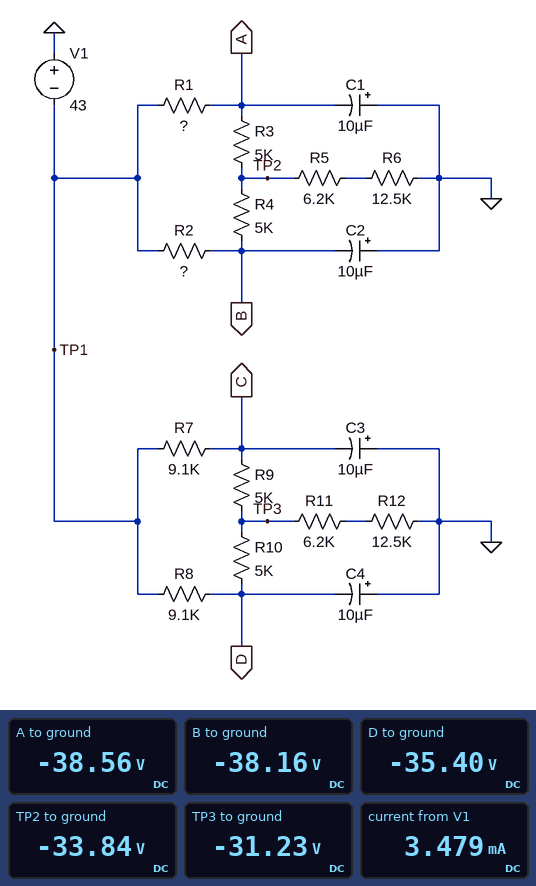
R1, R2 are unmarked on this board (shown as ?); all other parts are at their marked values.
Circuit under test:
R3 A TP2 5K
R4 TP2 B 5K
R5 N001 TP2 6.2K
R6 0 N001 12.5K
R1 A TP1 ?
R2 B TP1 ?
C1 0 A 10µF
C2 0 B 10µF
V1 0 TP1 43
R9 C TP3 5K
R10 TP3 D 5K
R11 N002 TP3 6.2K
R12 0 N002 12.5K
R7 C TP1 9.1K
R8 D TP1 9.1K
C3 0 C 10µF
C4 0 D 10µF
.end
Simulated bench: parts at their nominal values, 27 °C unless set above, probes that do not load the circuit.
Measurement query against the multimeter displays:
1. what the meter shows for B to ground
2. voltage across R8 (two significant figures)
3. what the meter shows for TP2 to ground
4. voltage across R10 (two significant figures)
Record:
-38.16 V
7.6 V
-33.84 V
4.2 V
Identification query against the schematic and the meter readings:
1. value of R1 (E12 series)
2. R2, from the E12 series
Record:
4.7 kΩ
5.6 kΩ
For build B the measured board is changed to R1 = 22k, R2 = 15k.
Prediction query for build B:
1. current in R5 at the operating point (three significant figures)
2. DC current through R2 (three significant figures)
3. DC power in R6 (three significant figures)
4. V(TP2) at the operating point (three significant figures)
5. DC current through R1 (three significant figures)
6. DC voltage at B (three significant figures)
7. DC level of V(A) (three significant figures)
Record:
1.42 mA
818 µA
25.4 mW
-26.6 V
606 µA
-30.7 V
-29.7 V
